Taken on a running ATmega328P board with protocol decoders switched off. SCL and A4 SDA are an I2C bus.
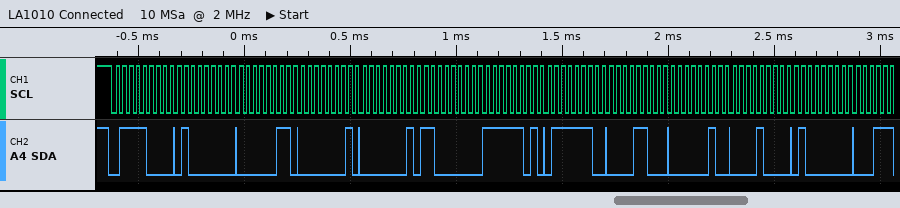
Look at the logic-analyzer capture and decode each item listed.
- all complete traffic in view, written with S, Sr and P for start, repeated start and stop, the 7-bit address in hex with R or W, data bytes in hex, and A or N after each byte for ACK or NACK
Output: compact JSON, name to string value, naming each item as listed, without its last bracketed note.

{"all complete traffic in view, written with S, Sr and P for start, repeated start and stop, the 7-bit address in hex with R or W, data bytes in hex, and A or N after each byte for ACK or NACK": "S 3CW A 40 A 03 A 01 A 01 A C0 A FD A 7E A 0C A 02 A 08 A 40 A"}
